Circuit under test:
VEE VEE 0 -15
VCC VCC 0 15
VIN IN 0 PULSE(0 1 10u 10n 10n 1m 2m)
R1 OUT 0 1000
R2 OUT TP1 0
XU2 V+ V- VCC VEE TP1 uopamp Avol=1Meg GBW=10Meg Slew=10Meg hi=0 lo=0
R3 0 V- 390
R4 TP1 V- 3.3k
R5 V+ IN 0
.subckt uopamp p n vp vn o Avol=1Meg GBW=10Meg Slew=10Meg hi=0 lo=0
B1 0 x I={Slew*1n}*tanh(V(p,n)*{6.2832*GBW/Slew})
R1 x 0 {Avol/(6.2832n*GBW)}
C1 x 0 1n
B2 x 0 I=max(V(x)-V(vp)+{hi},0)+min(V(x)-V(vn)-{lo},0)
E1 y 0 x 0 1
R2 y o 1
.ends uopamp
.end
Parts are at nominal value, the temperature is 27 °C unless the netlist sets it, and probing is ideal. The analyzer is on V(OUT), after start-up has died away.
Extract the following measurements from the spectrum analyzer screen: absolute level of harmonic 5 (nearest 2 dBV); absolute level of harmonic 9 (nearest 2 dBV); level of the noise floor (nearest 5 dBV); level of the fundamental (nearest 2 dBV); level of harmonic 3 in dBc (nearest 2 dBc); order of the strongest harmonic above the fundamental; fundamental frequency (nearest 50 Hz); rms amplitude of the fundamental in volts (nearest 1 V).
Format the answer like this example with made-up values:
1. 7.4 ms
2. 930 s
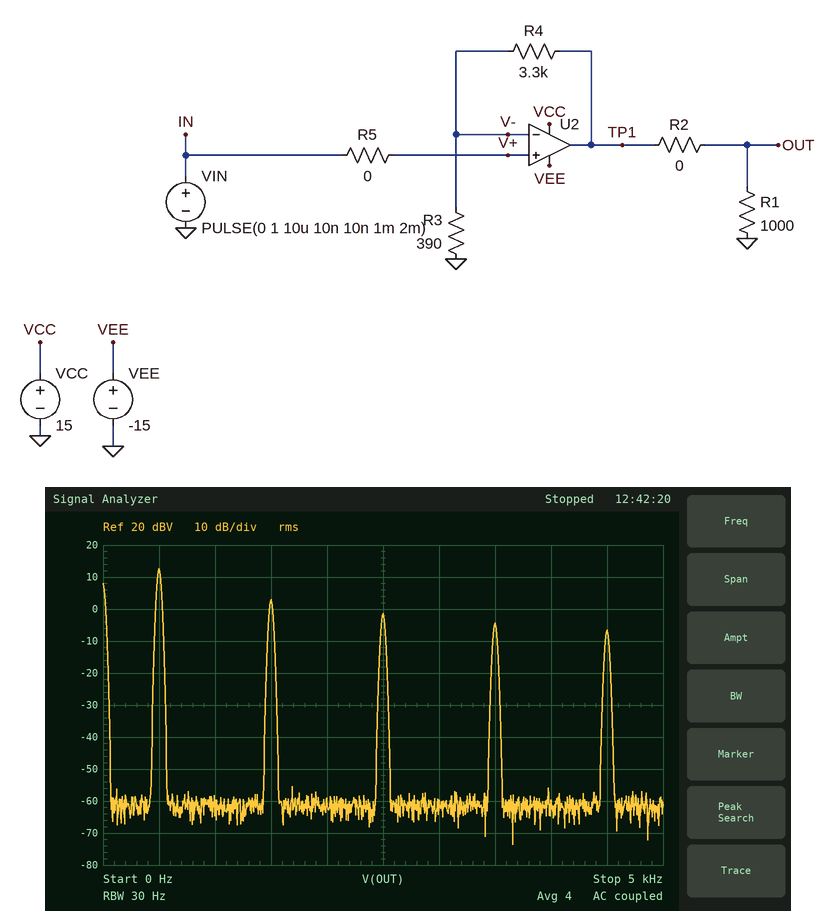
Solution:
1. -2 dBV
2. -6 dBV
3. -60 dBV
4. 12 dBV
5. -10 dBc
6. 3
7. 500 Hz
8. 4 V
